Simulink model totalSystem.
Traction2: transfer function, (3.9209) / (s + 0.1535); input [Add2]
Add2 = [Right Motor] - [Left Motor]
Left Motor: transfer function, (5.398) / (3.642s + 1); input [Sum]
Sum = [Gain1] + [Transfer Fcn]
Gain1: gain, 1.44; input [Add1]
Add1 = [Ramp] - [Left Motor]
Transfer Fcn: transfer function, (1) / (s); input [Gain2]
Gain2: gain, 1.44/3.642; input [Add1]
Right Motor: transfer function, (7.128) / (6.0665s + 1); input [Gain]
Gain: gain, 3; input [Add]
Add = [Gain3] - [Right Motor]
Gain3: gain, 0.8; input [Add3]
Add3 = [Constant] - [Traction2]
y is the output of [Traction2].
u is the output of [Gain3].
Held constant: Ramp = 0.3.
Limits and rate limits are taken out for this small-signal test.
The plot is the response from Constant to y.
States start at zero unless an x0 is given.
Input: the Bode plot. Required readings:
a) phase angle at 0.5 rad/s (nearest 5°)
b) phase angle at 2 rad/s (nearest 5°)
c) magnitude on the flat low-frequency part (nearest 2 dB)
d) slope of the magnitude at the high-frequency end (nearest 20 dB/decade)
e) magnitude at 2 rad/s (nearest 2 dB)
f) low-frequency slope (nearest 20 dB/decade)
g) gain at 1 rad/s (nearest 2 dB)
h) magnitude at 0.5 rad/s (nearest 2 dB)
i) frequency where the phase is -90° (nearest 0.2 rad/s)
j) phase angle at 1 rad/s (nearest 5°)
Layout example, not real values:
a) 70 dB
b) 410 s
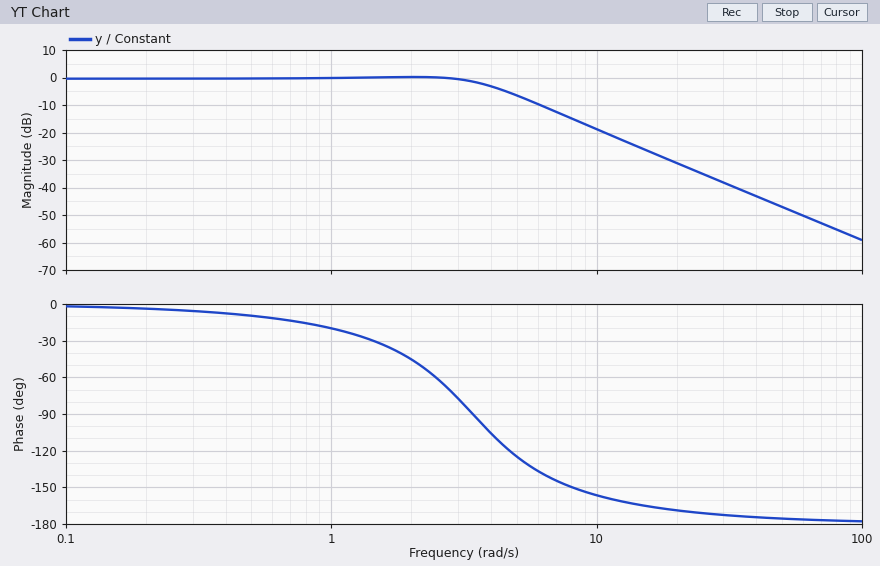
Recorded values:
a) -10°
b) -45°
c) 0 dB
d) -40 dB/decade
e) 0 dB
f) 0 dB/decade
g) 0 dB
h) 0 dB
i) 3.4 rad/s
j) -20°
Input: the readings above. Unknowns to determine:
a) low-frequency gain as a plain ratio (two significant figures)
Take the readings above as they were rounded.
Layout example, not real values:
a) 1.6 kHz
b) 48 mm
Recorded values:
a) 1.0
